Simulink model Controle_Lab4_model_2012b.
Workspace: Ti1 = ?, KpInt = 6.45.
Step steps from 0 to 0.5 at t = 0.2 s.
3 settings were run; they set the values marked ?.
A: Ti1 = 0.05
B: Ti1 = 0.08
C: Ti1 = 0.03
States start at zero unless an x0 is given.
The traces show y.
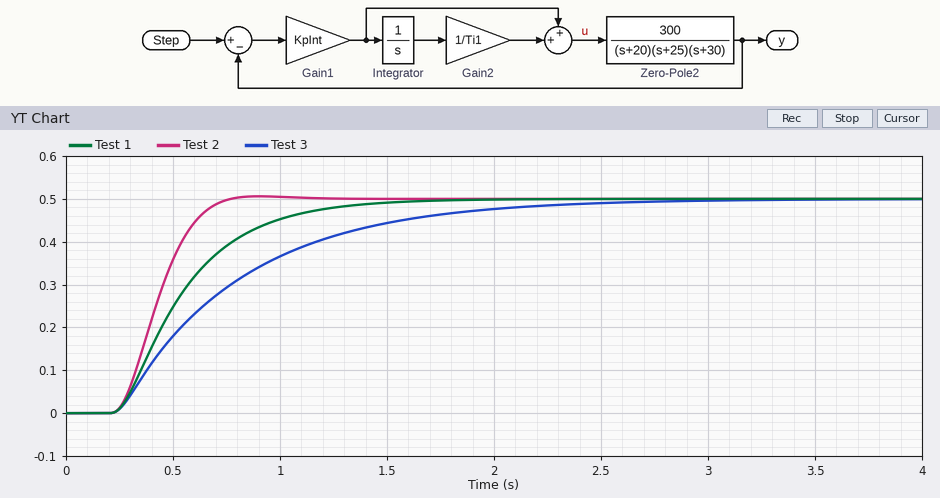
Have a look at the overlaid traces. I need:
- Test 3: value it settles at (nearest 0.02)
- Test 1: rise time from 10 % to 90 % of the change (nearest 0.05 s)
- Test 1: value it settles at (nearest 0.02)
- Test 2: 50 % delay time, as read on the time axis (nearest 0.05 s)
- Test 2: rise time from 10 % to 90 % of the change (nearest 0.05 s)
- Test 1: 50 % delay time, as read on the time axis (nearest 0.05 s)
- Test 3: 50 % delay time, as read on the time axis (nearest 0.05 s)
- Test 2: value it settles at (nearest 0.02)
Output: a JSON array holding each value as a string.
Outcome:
["0.50", "0.70 s", "0.50", "0.40 s", "0.30 s", "0.50 s", "0.65 s", "0.50"]
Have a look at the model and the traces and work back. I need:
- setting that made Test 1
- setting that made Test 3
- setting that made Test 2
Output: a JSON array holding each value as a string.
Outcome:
["A", "B", "C"]
